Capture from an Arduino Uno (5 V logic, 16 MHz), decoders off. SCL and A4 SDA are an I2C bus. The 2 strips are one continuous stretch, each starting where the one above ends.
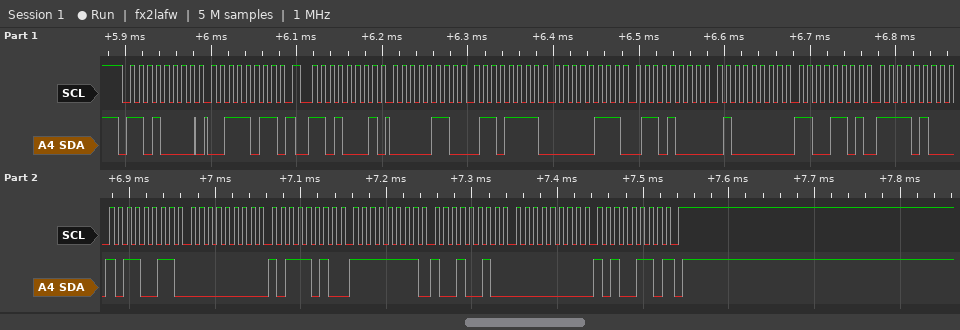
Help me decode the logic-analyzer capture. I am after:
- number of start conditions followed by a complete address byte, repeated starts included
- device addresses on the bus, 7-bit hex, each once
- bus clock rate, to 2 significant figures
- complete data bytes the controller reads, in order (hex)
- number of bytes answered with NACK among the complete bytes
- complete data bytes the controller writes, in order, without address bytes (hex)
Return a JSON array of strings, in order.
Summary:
["2", "0x68", "100 kHz", "06 6F 07 68 40 CD F4 B3 00 BA FF 92 00 A6", "1", "3B"]
